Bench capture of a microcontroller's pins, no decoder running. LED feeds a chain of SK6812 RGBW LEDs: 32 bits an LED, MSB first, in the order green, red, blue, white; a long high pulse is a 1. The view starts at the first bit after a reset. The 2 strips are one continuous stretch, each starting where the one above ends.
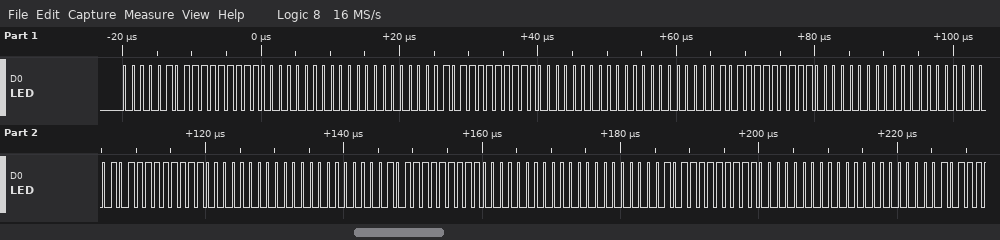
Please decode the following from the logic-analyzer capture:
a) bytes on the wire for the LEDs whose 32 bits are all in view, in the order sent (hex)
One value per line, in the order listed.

05 FF 00 00 05 FF 00 00 05 FF 00 00 05 FF 00 00 05 FF 00 00 05 FF 00 00
